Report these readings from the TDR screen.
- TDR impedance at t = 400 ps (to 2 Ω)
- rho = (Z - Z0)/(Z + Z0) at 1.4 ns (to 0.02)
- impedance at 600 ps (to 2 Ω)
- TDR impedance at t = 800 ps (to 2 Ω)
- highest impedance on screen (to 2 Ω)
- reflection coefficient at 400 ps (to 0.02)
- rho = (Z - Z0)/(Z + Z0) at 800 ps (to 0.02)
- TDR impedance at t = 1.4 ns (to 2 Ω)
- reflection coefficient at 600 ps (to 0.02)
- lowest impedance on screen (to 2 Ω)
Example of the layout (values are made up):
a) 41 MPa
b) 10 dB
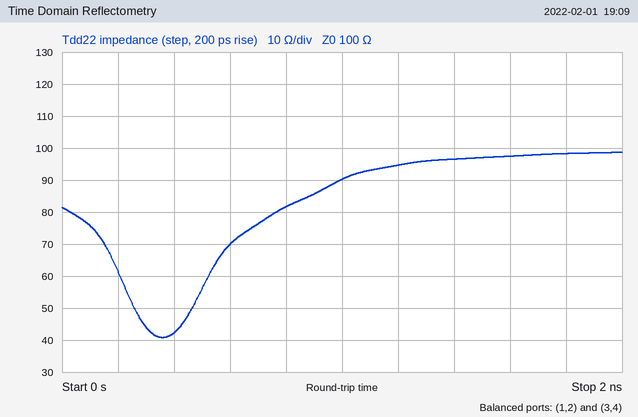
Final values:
a) 42 Ω
b) -0.02
c) 70 Ω
d) 82 Ω
e) 98 Ω
f) -0.40
g) -0.10
h) 96 Ω
i) -0.18
j) 40 Ω
